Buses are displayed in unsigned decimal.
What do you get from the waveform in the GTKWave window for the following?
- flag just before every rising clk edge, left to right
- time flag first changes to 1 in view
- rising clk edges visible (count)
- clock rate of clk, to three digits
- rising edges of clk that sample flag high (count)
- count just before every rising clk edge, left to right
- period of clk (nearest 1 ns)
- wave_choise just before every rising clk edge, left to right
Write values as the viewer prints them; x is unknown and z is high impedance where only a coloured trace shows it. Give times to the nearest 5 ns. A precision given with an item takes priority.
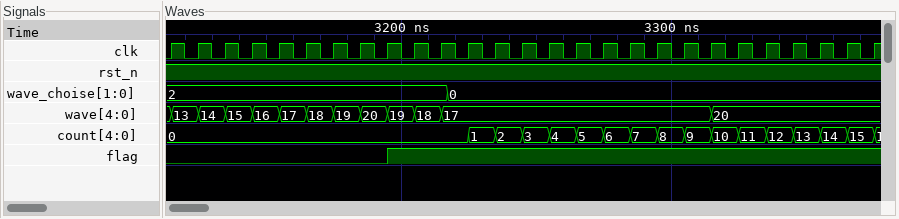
0 0 0 0 0 0 0 0 0 1 1 1 1 1 1 1 1 1 1 1 1 1 1 1 1 1 1
3195 ns
27
100 MHz
18
0, 0, 0, 0, 0, 0, 0, 0, 0, 0, 0, 0, 1, 2, 3, 4, 5, 6, 7, 8, 9, 10, 11, 12, 13, 14, 15
10 ns
2, 2, 2, 2, 2, 2, 2, 2, 2, 2, 2, 0, 0, 0, 0, 0, 0, 0, 0, 0, 0, 0, 0, 0, 0, 0, 0
